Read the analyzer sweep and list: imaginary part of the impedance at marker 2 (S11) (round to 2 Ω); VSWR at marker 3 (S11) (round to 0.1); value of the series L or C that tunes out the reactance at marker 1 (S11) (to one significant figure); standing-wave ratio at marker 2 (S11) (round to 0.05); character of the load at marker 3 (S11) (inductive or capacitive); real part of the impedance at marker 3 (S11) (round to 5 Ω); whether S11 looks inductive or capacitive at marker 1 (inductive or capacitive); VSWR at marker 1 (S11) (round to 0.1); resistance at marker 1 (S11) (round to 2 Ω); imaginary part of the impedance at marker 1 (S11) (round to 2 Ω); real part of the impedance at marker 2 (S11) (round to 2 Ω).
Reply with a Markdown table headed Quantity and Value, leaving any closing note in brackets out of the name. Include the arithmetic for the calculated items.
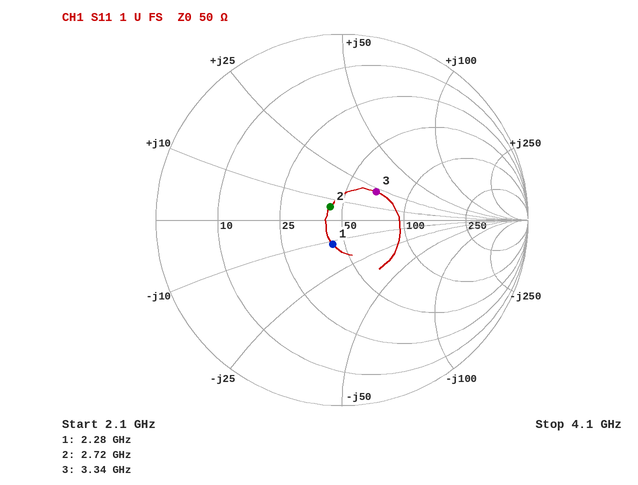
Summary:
| Quantity | Value |
|---|---|
| imaginary part of the impedance at marker 2 (S11) | +6 Ω |
| VSWR at marker 3 (S11) | 1.6 |
| value of the series L or C that tunes out the reactance at marker 1 (S11) | L = 12 Ω/(2π × 2.28 GHz) ≈ 838 pH, so 800 pH to one significant figure |
| standing-wave ratio at marker 2 (S11) | 1.20 |
| character of the load at marker 3 (S11) | inductive |
| real part of the impedance at marker 3 (S11) | 70 Ω |
| whether S11 looks inductive or capacitive at marker 1 | capacitive |
| VSWR at marker 1 (S11) | 1.3 |
| resistance at marker 1 (S11) | 44 Ω |
| imaginary part of the impedance at marker 1 (S11) | -12 Ω |
| real part of the impedance at marker 2 (S11) | 44 Ω |
